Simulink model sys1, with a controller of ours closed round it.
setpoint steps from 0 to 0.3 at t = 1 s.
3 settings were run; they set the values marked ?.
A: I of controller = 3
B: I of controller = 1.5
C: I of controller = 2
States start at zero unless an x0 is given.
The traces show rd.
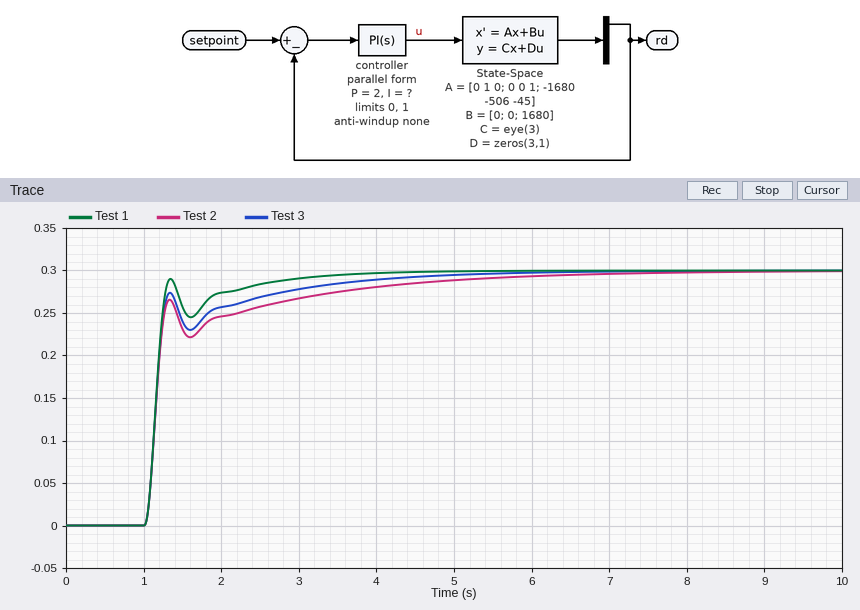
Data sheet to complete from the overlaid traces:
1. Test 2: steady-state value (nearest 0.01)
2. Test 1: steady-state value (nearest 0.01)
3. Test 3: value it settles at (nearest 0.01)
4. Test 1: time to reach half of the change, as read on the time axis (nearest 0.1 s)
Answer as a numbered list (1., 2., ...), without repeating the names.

1. 0.30
2. 0.30
3. 0.30
4. 1.2 s
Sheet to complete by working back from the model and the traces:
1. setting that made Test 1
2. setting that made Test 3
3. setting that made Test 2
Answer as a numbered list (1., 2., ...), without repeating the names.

1. A
2. C
3. B
